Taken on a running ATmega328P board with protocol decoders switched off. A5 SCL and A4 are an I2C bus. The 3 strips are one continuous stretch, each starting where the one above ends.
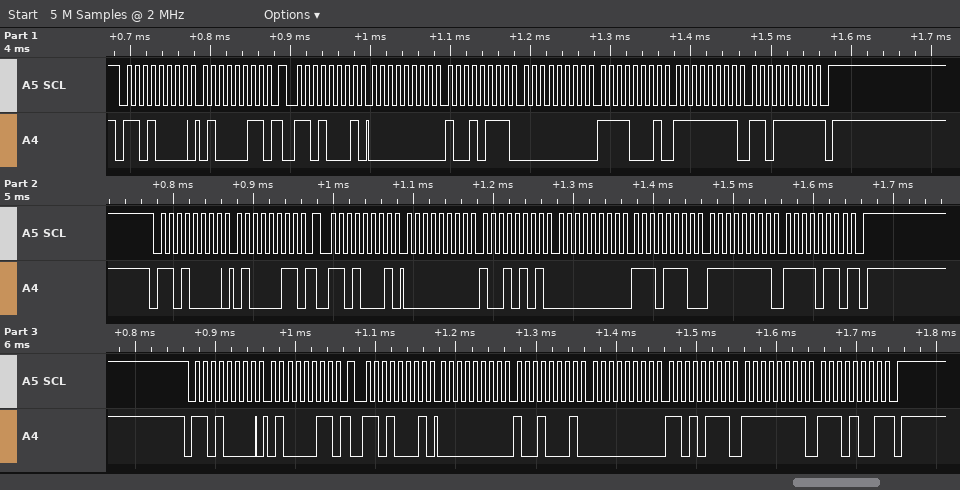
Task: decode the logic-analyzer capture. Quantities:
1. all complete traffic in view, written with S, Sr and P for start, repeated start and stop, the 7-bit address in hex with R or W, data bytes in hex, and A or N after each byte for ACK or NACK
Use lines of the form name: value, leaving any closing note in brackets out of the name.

all complete traffic in view, written with S, Sr and P for start, repeated start and stop, the 7-bit address in hex with R or W, data bytes in hex, and A or N after each byte for ACK or NACK: S 68W A 43 A Sr 68R A 00 A 97 A 00 A F1 A FF A DF N P S 68W A 43 A Sr 68R A 00 A 95 A 00 A EE A FF A F6 N P S 68W A 43 A Sr 68R A 00 A 91 A 00 A D7 A FF A E9 N P
